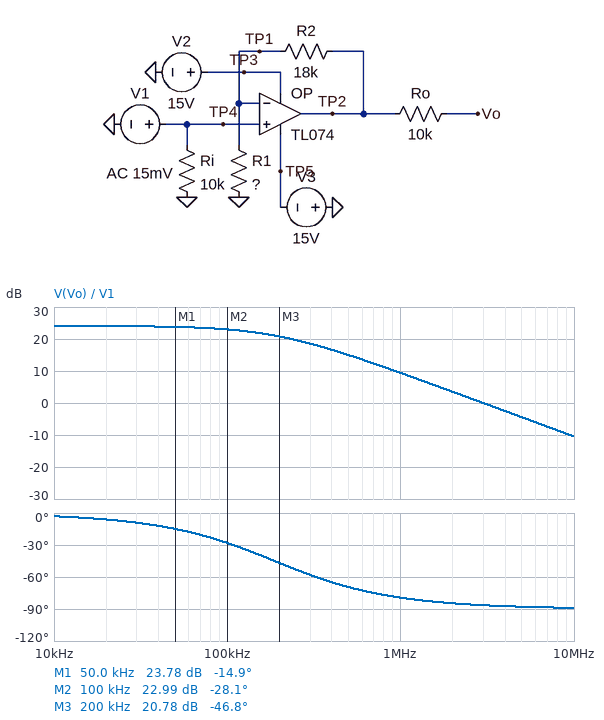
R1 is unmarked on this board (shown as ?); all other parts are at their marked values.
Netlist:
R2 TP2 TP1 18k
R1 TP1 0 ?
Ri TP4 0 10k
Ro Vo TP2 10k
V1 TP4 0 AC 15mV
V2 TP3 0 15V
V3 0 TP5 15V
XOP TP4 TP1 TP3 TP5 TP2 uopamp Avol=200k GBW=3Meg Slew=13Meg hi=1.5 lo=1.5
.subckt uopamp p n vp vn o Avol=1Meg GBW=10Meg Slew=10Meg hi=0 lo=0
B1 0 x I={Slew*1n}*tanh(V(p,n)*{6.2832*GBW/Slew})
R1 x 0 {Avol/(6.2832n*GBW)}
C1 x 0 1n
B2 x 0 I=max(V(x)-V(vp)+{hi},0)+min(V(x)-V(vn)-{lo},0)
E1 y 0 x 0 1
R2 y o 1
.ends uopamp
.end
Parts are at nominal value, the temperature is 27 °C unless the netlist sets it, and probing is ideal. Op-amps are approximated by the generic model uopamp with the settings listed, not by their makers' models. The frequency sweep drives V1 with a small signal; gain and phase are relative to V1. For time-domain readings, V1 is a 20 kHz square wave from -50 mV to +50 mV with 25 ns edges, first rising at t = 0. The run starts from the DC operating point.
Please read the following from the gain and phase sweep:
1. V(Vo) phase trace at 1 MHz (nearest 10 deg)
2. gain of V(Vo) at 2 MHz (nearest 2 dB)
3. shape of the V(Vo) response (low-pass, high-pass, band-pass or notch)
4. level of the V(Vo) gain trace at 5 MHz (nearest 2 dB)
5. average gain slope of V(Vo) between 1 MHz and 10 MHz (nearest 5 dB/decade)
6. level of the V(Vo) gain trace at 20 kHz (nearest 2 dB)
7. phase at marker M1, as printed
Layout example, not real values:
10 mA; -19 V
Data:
-80 deg; 4 dB; low-pass; -4 dB; -20 dB/decade; 24 dB; -14.9 deg
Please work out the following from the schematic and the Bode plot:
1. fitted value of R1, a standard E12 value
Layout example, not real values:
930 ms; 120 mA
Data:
1.2 kΩ
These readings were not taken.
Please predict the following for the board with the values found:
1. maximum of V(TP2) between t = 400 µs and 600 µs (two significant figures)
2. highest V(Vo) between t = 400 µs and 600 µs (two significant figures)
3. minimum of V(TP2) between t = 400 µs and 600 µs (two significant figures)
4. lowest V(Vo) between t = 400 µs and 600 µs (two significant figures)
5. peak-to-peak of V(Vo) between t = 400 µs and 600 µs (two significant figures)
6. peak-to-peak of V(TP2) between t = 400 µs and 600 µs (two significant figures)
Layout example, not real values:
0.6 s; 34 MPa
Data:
800 mV; 800 mV; -800 mV; -800 mV; 1.6 V; 1.6 V
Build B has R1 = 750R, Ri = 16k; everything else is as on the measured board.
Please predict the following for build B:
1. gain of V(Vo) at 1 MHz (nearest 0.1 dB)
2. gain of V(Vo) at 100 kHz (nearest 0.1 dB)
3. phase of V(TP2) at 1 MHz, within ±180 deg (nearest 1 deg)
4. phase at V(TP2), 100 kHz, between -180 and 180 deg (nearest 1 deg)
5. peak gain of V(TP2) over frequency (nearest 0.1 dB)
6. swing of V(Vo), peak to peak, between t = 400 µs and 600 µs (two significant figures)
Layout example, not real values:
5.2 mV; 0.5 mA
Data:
9.5 dB; 25.7 dB; -83 deg; -40 deg; 28.0 dB; 2.5 V
